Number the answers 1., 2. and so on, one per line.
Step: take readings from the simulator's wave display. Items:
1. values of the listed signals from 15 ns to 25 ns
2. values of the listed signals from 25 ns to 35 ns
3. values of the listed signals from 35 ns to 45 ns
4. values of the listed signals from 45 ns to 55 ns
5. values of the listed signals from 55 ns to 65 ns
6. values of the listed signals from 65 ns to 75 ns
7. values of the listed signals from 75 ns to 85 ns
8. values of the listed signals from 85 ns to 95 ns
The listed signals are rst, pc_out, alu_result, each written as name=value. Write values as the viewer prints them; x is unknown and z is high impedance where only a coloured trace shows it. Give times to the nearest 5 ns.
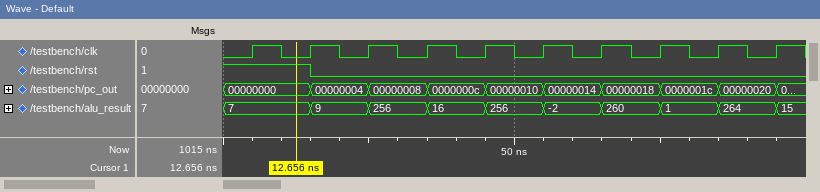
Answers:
1. rst=0, pc_out=00000004, alu_result=9
2. rst=0, pc_out=00000008, alu_result=256
3. rst=0, pc_out=0000000c, alu_result=16
4. rst=0, pc_out=00000010, alu_result=256
5. rst=0, pc_out=00000014, alu_result=-2
6. rst=0, pc_out=00000018, alu_result=260
7. rst=0, pc_out=0000001c, alu_result=1
8. rst=0, pc_out=00000020, alu_result=264
